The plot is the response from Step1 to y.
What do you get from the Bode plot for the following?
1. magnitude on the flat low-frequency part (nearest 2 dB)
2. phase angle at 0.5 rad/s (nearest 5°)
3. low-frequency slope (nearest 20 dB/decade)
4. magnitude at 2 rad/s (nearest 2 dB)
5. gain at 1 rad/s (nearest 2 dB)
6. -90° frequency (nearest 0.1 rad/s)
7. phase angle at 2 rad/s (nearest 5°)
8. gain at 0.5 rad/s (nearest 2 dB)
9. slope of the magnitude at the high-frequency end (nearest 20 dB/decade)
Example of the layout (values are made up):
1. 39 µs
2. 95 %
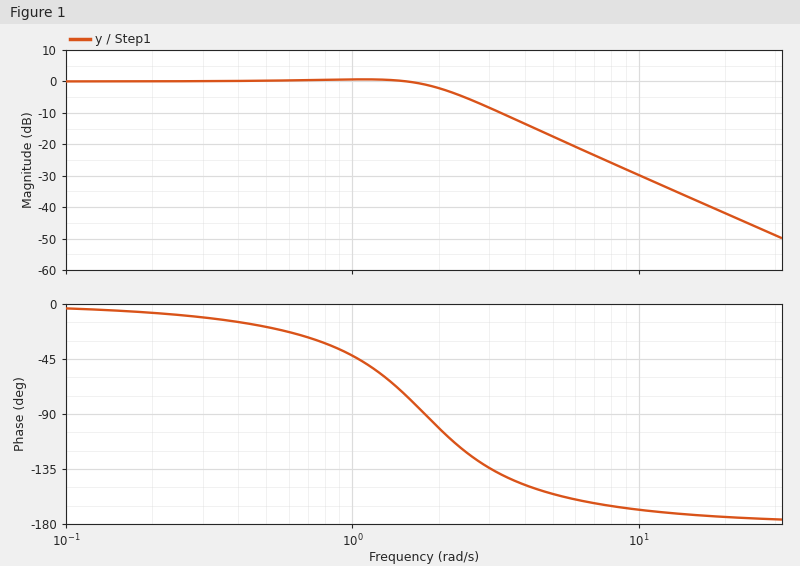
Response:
1. 0 dB
2. -20°
3. 0 dB/decade
4. -2 dB
5. 0 dB
6. 1.8 rad/s
7. -100°
8. 0 dB
9. -40 dB/decade
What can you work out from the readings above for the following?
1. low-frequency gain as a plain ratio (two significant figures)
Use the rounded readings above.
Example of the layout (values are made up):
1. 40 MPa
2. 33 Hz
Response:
1. 1.0
